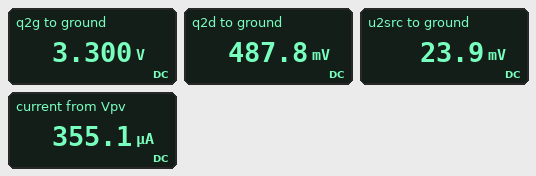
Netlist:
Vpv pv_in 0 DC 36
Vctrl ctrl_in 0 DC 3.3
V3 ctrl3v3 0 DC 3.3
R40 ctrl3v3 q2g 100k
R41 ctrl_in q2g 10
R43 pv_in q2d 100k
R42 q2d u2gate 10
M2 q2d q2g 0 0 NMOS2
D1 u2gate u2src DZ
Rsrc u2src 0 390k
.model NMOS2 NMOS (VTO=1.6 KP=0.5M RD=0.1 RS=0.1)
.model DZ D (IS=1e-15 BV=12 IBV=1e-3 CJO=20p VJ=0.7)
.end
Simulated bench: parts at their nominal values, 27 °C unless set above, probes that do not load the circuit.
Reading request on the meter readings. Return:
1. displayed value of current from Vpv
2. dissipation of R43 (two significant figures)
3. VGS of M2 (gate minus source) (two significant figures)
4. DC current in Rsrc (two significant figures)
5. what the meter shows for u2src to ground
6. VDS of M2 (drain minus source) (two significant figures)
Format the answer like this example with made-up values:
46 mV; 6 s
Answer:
355.1 µA; 13 mW; 3.3 V; 61 nA; 23.9 mV; 490 mV
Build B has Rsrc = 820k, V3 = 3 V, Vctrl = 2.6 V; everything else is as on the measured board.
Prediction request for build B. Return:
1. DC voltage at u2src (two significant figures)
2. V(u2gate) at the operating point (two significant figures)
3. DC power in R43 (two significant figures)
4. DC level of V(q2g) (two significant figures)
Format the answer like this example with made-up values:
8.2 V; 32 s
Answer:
9.3 V; 9.9 V; 6.8 mW; 2.6 V
